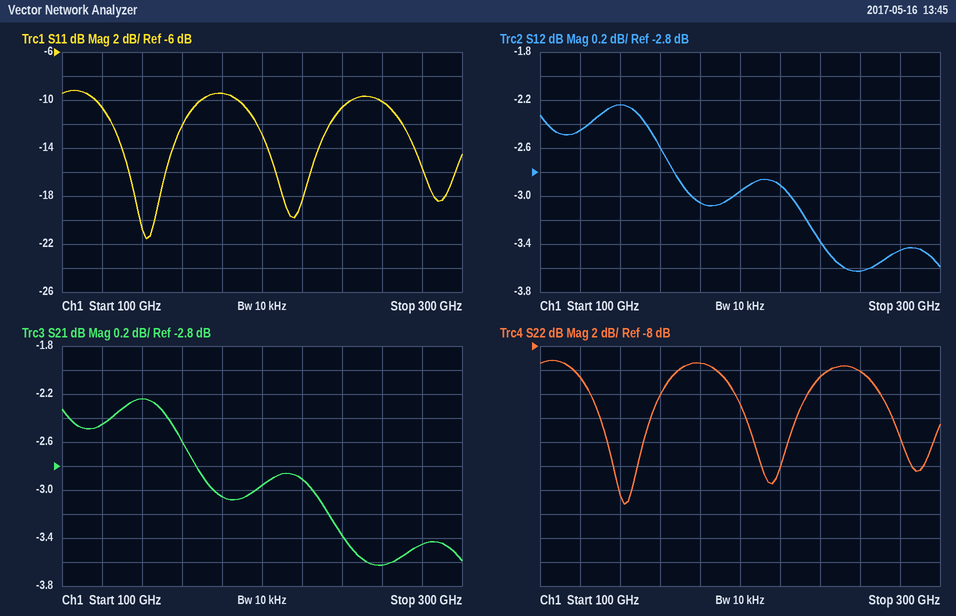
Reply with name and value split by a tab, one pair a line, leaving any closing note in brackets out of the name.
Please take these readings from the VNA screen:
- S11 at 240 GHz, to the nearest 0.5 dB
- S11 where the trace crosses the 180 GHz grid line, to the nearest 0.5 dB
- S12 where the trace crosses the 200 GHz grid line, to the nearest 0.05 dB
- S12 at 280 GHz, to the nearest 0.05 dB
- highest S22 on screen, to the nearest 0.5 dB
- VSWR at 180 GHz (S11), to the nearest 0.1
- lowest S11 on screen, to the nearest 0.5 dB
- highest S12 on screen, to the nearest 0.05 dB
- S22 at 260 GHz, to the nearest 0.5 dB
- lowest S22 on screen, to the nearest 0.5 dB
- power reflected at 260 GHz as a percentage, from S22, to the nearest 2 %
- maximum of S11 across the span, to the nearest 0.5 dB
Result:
S11 at 240 GHz, to the nearest 0.5 dB	-10.5 dB
S11 where the trace crosses the 180 GHz grid line, to the nearest 0.5 dB	-9.5 dB
S12 where the trace crosses the 200 GHz grid line, to the nearest 0.05 dB	-2.95 dB
S12 at 280 GHz, to the nearest 0.05 dB	-3.45 dB
highest S22 on screen, to the nearest 0.5 dB	-9.0 dB
VSWR at 180 GHz (S11), to the nearest 0.1	2.0
lowest S11 on screen, to the nearest 0.5 dB	-21.5 dB
highest S12 on screen, to the nearest 0.05 dB	-2.25 dB
S22 at 260 GHz, to the nearest 0.5 dB	-10.0 dB
lowest S22 on screen, to the nearest 0.5 dB	-21.0 dB
power reflected at 260 GHz as a percentage, from S22, to the nearest 2 %	10 %
maximum of S11 across the span, to the nearest 0.5 dB	-9.0 dB
